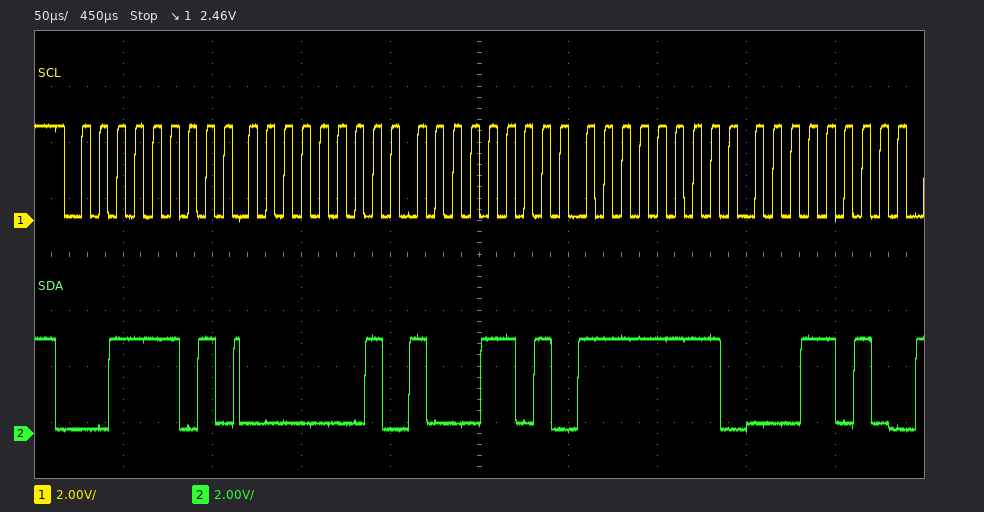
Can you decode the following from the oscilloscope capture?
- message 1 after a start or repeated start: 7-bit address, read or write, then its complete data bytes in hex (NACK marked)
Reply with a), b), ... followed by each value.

a) 0x1E read: 01 8D FF 1A
